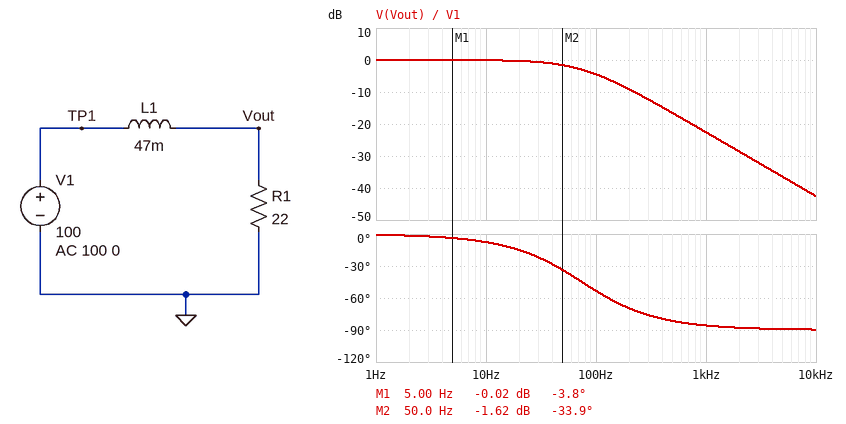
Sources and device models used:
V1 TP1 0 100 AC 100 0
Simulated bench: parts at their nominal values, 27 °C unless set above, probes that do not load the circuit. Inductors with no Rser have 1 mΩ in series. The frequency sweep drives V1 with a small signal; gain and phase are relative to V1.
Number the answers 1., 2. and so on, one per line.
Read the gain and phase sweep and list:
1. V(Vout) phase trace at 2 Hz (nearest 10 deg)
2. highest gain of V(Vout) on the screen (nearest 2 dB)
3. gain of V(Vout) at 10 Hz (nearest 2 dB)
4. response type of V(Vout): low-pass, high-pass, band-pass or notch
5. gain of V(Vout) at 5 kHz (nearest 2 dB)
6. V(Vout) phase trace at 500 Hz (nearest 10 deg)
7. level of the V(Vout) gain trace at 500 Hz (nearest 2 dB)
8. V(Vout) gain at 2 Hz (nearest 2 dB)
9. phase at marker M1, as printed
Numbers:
1. 0 deg
2. 0 dB
3. 0 dB
4. low-pass
5. -36 dB
6. -80 deg
7. -16 dB
8. 0 dB
9. -3.8 deg
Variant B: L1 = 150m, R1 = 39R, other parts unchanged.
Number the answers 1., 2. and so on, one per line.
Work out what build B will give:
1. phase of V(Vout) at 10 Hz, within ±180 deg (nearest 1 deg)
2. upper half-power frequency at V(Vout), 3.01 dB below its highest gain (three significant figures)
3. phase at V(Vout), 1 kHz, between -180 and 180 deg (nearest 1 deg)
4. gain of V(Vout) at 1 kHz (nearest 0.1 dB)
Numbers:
1. -14 deg
2. 41.4 Hz
3. -88 deg
4. -27.7 dB
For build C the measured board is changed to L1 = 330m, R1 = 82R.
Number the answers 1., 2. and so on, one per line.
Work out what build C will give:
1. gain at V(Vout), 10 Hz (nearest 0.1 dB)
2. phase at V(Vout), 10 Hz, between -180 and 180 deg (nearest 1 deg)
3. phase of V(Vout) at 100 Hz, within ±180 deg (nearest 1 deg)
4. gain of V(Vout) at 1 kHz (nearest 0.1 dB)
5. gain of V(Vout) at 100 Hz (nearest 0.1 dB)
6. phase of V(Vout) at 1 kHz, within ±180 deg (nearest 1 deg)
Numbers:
1. -0.3 dB
2. -14 deg
3. -68 deg
4. -28.1 dB
5. -8.7 dB
6. -88 deg
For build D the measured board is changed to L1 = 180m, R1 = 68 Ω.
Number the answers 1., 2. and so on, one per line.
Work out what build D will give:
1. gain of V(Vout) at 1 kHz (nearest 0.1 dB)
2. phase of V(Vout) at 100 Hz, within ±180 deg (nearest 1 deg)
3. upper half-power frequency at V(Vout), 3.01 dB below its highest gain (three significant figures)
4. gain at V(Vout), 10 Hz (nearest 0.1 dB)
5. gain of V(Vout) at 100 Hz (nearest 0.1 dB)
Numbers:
1. -24.4 dB
2. -59 deg
3. 60.1 Hz
4. -0.1 dB
5. -5.8 dB
